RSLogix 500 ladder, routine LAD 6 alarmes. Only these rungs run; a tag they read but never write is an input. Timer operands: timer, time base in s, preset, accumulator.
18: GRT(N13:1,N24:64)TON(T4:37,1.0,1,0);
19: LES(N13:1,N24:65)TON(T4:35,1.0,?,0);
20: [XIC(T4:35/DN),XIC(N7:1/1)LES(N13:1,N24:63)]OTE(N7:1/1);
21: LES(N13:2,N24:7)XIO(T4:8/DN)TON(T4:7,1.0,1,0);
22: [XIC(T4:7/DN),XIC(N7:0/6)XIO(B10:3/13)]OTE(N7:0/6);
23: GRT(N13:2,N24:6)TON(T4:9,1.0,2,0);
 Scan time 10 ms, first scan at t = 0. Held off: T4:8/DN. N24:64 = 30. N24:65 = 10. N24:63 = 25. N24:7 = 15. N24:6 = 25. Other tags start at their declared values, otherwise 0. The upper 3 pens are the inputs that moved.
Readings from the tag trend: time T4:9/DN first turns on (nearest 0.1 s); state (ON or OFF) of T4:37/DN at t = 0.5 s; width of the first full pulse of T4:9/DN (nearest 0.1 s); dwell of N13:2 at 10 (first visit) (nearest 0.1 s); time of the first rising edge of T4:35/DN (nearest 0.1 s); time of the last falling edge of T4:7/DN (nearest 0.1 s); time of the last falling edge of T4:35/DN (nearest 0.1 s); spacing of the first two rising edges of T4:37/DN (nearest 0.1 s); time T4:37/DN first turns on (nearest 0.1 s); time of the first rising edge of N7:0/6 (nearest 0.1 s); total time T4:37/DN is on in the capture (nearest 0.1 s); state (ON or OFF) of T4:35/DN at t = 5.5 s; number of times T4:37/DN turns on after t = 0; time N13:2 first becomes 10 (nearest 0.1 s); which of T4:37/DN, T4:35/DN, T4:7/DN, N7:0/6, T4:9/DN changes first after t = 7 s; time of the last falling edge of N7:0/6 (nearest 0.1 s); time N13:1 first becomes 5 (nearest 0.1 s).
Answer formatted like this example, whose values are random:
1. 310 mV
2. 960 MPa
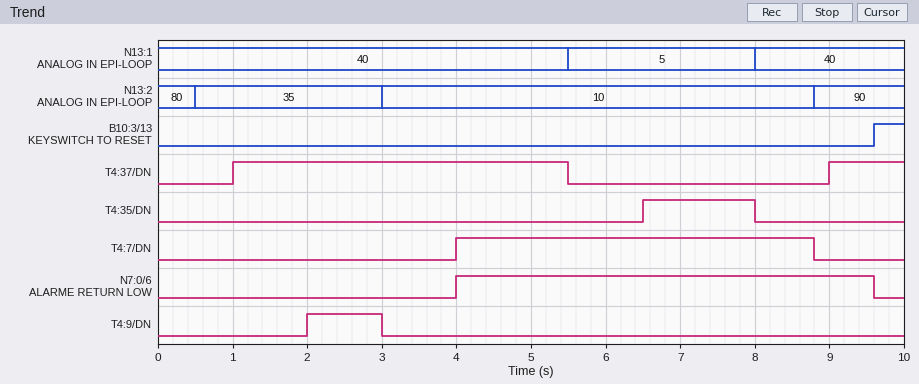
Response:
1. 2.0 s
2. OFF
3. 1.0 s
4. 5.8 s
5. 6.5 s
6. 8.8 s
7. 8.0 s
8. 8.0 s
9. 1.0 s
10. 4.0 s
11. 5.5 s
12. OFF
13. 2
14. 3.0 s
15. T4:35/DN
16. 9.6 s
17. 5.5 s
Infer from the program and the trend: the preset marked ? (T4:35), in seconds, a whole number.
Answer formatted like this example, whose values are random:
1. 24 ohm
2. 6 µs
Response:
1. 1 s
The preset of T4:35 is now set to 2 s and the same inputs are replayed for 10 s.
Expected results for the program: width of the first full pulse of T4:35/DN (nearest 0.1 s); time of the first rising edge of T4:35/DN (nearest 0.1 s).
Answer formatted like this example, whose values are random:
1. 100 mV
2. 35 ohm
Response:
1. 0.5 s
2. 7.5 s
